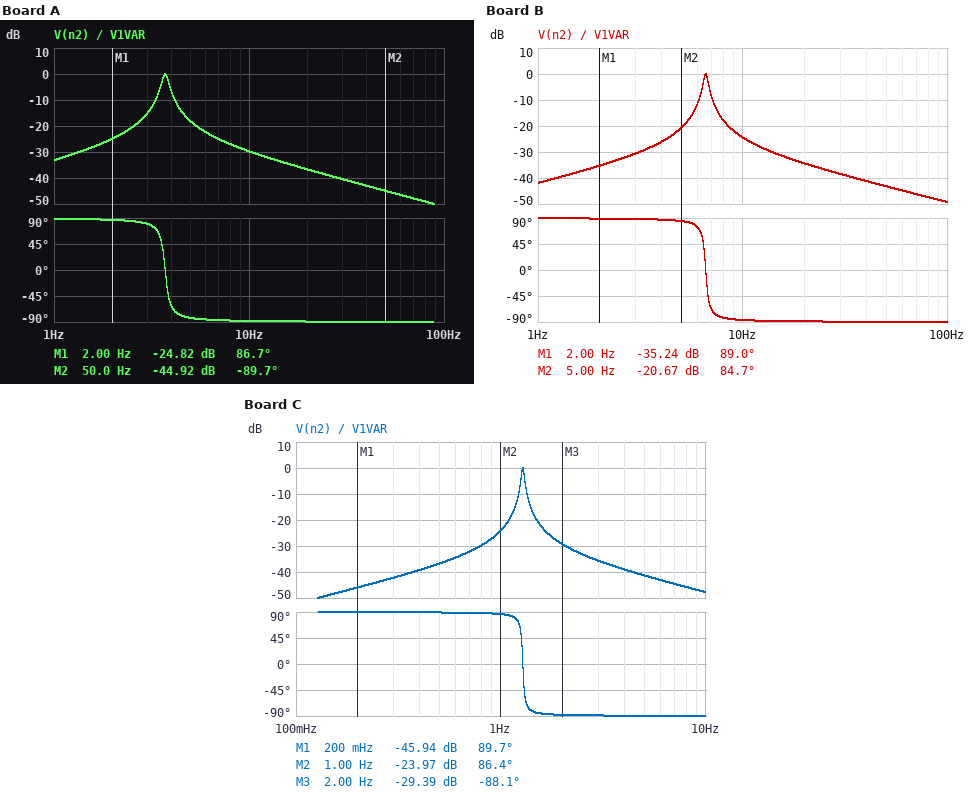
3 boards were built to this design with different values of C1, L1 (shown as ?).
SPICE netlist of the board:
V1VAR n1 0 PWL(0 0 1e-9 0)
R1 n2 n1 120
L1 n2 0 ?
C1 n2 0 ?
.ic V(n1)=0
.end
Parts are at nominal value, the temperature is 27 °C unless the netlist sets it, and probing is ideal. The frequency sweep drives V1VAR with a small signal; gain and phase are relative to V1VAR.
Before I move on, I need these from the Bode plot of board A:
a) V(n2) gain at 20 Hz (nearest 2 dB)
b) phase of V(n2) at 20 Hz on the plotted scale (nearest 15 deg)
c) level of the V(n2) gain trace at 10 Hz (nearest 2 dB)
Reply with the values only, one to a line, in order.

-36 dB
-90 deg
-30 dB
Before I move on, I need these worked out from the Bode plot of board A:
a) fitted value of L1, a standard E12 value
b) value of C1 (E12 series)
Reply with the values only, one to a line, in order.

390 mH
4.7 mF
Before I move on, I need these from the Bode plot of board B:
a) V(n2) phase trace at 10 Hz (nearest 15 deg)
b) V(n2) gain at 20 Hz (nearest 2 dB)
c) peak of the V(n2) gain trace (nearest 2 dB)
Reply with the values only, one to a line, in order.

-90 deg
-34 dB
0 dB
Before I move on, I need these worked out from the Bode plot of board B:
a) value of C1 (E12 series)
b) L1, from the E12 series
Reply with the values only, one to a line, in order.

3.9 mF
150 mH
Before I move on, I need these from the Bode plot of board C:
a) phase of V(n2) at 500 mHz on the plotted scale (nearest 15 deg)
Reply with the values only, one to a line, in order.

90 deg
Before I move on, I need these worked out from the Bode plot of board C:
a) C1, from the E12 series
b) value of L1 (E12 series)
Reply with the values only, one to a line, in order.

33 mF
470 mH
